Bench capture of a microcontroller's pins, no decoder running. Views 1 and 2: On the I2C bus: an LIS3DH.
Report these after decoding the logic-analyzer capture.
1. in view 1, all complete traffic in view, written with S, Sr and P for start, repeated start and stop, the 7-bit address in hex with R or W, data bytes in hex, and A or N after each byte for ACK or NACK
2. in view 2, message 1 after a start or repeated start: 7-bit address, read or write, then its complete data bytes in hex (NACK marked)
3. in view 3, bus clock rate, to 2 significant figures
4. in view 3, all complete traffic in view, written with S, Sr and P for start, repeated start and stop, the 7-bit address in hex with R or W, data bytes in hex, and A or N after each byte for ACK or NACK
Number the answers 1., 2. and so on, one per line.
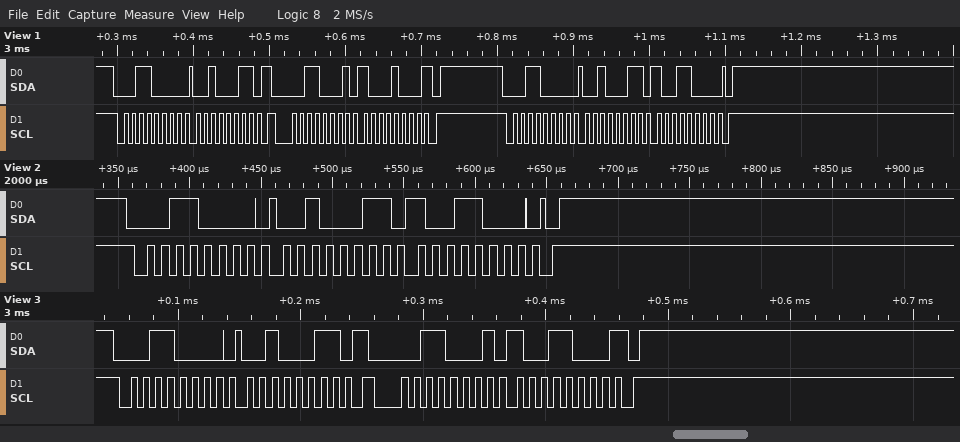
1. S 18W A 23 A Sr 18R A 88 N P S 18W A 23 A 98 A P
2. 0x18 write: 23 98
3. 100 kHz
4. S 18W A 23 A Sr 18R A 98 N P
